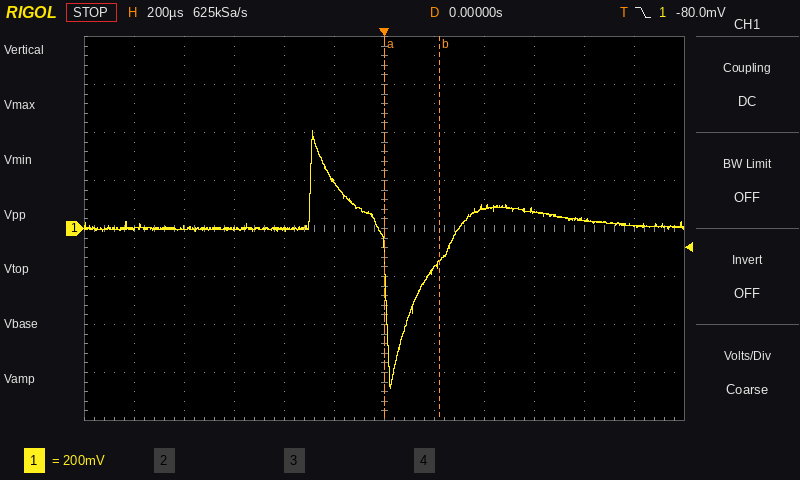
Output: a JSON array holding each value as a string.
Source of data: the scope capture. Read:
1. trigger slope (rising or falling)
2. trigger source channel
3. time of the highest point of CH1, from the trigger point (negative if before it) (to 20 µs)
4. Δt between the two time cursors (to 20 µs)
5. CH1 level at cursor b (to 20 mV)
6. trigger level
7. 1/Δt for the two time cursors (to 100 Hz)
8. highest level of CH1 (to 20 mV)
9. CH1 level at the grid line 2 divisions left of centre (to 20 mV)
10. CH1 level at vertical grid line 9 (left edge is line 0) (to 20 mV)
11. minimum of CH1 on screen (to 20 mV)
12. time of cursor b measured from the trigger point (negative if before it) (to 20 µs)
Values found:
["falling", "CH1", "-280 µs", "220 µs", "-140 mV", "-80.0 mV", "4.5 kHz", "400 mV", "0 mV", "80 mV", "-660 mV", "+220 µs"]
